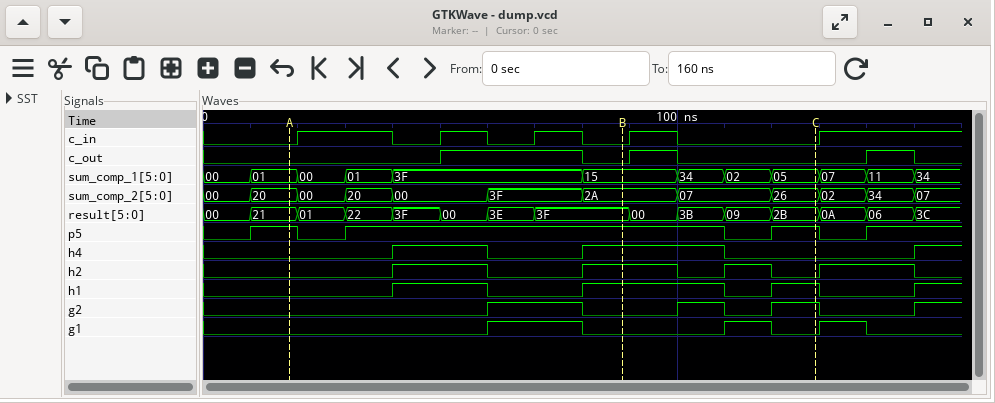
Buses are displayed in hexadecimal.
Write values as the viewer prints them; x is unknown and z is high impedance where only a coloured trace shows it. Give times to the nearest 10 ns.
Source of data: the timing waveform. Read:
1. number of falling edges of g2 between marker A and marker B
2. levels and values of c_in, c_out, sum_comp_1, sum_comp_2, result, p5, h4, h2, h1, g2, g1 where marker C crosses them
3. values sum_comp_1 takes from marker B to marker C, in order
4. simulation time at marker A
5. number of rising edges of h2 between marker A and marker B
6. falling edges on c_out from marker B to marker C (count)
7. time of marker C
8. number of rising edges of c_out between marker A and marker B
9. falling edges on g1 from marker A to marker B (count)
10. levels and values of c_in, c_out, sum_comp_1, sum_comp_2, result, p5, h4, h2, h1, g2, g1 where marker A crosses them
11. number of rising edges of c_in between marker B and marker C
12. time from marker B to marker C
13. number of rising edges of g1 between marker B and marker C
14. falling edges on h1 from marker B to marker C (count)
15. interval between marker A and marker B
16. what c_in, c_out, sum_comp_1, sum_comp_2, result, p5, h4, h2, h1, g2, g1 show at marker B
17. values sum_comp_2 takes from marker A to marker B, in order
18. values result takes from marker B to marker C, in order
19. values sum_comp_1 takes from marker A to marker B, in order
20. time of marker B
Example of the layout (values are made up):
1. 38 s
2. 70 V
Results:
1. 1
2. c_in=0, c_out=0, sum_comp_1=05, sum_comp_2=26, result=2B, p5=1, h4=0, h2=0, h1=1, g2=1, g1=0
3. 15, 34, 02, 05
4. 20 ns
5. 2
6. 1
7. 130 ns
8. 1
9. 1
10. c_in=0, c_out=0, sum_comp_1=01, sum_comp_2=20, result=21, p5=1, h4=0, h2=0, h1=0, g2=0, g1=0
11. 1
12. 40 ns
13. 1
14. 1
15. 70 ns
16. c_in=0, c_out=0, sum_comp_1=15, sum_comp_2=2A, result=3F, p5=1, h4=1, h2=1, h1=1, g2=0, g1=0
17. 20, 00, 20, 00, 3F, 2A
18. 3F, 00, 3B, 09, 2B
19. 01, 00, 01, 3F, 15
20. 90 ns
